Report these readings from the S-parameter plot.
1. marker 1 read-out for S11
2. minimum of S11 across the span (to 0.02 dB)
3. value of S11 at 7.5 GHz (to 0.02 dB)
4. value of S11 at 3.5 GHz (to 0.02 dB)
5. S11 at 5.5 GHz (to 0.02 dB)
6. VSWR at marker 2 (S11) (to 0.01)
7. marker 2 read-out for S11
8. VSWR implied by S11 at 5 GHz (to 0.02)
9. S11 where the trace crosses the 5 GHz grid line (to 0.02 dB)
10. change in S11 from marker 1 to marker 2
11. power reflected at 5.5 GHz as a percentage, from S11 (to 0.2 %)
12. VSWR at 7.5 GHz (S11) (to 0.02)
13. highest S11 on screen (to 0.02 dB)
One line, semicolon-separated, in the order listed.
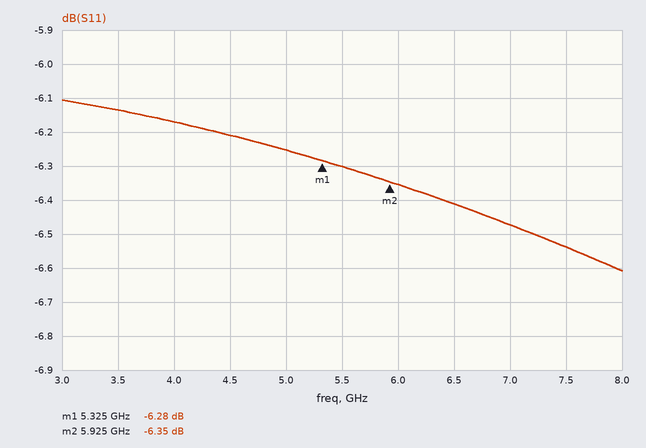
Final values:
-6.28 dB; -6.60 dB; -6.54 dB; -6.14 dB; -6.30 dB; 2.86; -6.35 dB; 2.90; -6.26 dB; -0.07 dB; 23.4 %; 2.78; -6.10 dB
